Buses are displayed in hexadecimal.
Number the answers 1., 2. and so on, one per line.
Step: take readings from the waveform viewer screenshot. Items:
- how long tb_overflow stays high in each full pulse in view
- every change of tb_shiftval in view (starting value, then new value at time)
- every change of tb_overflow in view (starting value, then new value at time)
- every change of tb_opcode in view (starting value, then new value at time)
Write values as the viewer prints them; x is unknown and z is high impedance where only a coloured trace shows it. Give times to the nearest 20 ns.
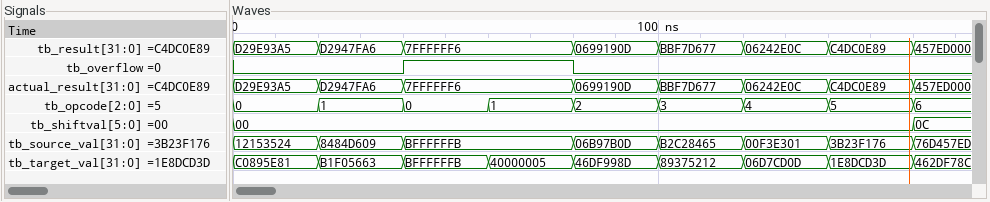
1. 40 ns
2. 00, 0C at 160 ns
3. 0, 1 at 40 ns, 0 at 80 ns
4. 0, 1 at 20 ns, 0 at 40 ns, 1 at 60 ns, 2 at 80 ns, 3 at 100 ns, 4 at 120 ns, 5 at 140 ns, 6 at 160 ns
